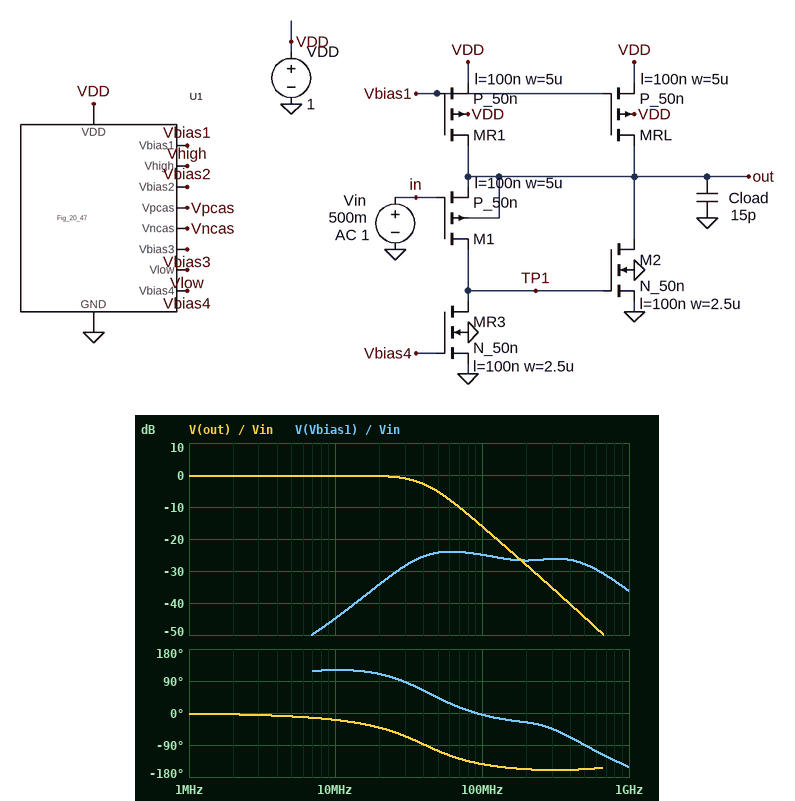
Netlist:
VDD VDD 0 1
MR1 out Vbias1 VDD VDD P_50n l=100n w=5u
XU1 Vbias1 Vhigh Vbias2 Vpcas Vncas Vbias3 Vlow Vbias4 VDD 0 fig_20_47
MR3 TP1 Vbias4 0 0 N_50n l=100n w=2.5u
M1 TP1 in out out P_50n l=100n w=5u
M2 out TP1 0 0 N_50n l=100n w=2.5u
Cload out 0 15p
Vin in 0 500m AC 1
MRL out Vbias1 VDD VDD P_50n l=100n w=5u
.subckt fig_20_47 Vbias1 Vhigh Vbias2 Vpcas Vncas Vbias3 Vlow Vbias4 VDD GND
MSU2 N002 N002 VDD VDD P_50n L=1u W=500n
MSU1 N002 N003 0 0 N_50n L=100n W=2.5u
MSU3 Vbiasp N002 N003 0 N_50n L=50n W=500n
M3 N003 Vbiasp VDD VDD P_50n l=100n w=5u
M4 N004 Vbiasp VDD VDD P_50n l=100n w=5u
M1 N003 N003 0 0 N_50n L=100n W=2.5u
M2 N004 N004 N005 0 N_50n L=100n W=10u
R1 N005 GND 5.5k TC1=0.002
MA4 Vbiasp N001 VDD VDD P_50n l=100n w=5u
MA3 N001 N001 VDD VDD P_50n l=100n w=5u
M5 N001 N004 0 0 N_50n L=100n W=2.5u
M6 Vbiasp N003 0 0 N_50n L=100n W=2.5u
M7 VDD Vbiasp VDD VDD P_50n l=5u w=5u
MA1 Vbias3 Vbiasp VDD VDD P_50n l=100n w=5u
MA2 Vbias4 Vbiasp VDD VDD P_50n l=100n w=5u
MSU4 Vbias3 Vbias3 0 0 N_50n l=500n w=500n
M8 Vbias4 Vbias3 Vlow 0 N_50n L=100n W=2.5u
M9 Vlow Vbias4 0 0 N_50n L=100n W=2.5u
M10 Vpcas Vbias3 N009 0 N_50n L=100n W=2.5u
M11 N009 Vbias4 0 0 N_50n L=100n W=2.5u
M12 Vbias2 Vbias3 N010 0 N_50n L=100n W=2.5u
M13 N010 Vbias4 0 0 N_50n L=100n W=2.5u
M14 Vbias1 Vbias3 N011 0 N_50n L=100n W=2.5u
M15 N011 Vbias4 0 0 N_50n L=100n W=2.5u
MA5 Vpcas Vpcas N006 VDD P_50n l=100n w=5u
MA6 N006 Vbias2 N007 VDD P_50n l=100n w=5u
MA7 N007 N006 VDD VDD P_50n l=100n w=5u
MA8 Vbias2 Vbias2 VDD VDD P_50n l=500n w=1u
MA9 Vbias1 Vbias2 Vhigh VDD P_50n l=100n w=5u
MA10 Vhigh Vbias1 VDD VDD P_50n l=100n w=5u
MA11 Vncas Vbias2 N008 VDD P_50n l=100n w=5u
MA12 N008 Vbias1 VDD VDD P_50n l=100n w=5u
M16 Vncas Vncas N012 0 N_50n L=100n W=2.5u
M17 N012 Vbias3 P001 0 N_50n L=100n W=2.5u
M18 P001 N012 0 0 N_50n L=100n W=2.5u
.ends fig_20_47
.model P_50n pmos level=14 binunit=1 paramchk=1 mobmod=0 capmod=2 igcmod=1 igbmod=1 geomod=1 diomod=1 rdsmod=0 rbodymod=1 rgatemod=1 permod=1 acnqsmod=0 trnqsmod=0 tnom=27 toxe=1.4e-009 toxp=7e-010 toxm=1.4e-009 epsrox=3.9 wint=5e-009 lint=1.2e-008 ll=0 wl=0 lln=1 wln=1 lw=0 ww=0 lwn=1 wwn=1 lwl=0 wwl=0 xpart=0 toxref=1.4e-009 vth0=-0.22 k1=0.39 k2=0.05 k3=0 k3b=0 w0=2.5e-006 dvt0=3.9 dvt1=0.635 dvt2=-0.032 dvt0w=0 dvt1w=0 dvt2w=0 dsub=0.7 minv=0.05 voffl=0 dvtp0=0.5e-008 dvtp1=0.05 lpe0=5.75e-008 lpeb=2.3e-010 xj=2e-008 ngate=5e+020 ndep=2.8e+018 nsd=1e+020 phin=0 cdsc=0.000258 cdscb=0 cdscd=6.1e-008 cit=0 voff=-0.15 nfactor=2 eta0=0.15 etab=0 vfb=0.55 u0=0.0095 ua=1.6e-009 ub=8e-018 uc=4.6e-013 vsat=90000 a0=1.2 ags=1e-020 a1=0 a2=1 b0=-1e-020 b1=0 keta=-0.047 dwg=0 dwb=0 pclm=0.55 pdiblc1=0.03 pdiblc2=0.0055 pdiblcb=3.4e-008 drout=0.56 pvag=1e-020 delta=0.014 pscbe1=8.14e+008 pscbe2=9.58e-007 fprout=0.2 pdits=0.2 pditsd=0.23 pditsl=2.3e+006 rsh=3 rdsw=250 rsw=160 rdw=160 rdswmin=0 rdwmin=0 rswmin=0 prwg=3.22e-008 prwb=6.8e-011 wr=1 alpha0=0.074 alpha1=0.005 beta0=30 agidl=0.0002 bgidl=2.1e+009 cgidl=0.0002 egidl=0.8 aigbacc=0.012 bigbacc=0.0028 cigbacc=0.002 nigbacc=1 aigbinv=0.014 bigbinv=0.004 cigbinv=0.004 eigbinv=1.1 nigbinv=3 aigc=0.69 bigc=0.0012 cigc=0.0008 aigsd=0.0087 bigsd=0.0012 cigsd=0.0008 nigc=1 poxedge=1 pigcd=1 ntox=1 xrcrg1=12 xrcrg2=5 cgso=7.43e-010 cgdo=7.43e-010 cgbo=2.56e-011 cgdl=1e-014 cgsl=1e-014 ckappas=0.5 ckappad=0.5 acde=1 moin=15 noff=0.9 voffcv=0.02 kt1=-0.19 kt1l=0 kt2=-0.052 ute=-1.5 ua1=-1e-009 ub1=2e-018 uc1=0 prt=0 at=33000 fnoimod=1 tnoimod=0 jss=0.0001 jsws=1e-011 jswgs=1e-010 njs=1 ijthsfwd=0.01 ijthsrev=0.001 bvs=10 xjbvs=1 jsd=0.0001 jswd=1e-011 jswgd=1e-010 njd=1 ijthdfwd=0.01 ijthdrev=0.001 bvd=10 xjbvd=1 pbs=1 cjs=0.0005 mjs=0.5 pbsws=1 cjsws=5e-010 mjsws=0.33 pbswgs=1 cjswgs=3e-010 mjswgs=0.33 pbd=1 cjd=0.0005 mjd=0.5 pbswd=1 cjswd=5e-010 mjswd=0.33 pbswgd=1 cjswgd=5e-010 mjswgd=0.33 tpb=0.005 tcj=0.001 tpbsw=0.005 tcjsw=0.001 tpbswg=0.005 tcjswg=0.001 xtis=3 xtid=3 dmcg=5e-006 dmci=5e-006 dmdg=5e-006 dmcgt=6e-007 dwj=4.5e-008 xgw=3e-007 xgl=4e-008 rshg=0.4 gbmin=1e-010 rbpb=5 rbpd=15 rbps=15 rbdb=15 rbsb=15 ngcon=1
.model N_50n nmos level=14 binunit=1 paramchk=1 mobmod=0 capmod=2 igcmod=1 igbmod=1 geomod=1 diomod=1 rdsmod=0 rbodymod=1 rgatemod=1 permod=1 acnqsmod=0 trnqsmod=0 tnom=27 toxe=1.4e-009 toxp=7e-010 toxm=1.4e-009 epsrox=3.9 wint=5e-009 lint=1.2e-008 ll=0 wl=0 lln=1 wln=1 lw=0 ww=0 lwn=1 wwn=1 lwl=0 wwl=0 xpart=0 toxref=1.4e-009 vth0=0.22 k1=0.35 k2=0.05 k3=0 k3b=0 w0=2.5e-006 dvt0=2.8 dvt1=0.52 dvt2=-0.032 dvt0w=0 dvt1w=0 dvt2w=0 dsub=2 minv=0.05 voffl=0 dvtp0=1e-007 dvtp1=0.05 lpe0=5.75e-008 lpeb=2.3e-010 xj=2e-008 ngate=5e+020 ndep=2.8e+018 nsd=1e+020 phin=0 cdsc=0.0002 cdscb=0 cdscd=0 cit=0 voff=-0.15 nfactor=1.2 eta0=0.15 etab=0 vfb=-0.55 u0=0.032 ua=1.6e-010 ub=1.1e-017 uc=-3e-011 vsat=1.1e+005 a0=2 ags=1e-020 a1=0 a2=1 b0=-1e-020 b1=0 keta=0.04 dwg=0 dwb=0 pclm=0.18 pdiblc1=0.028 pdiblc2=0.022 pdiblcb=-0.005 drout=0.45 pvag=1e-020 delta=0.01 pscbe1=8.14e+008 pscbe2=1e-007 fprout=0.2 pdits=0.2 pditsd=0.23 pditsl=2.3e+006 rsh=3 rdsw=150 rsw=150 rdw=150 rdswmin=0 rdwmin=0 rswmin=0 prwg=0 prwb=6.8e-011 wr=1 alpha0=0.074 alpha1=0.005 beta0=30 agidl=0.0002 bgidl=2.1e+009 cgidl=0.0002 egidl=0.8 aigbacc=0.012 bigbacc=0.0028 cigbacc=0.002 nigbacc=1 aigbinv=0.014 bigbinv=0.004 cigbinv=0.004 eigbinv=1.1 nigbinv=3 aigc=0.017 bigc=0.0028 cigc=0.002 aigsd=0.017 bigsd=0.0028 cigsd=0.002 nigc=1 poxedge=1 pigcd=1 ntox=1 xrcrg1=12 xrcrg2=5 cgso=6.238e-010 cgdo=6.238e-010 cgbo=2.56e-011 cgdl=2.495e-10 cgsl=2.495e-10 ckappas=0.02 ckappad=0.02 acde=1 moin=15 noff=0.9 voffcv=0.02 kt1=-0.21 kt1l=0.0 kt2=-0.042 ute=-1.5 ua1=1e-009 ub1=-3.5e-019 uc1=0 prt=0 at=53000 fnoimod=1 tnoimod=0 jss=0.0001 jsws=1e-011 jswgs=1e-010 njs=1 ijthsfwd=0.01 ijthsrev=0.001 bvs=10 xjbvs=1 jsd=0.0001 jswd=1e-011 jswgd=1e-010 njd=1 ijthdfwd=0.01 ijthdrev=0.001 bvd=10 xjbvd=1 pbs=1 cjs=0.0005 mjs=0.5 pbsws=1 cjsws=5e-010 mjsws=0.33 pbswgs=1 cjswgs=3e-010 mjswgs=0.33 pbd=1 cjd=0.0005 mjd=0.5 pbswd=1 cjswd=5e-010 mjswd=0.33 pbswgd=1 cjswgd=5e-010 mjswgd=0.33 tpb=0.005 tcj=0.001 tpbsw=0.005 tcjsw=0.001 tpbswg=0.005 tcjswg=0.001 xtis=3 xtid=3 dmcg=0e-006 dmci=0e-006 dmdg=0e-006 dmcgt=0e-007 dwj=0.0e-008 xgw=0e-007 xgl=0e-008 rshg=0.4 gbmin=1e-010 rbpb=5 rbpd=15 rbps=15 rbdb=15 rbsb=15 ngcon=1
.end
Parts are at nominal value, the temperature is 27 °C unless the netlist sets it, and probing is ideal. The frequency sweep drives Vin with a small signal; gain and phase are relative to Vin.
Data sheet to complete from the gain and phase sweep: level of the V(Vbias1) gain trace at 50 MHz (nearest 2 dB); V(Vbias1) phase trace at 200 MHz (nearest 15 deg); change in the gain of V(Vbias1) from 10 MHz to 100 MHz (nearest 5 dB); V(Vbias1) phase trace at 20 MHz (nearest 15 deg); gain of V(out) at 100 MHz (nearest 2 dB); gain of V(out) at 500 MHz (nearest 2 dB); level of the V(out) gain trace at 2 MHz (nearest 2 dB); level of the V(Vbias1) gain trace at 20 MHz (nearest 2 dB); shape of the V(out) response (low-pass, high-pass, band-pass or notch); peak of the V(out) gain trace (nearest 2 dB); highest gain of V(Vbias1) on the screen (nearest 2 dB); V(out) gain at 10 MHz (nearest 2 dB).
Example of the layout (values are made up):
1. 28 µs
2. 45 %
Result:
1. -24 dB
2. -30 deg
3. 20 dB
4. 105 deg
5. -16 dB
6. -44 dB
7. 0 dB
8. -34 dB
9. low-pass
10. 0 dB
11. -24 dB
12. 0 dB
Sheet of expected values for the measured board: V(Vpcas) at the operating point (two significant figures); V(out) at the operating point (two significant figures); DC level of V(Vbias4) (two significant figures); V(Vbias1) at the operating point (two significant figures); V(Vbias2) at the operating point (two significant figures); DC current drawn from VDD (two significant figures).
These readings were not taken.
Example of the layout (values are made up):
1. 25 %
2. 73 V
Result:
1. 200 mV
2. 860 mV
3. 360 mV
4. 640 mV
5. 370 mV
6. 130 µA
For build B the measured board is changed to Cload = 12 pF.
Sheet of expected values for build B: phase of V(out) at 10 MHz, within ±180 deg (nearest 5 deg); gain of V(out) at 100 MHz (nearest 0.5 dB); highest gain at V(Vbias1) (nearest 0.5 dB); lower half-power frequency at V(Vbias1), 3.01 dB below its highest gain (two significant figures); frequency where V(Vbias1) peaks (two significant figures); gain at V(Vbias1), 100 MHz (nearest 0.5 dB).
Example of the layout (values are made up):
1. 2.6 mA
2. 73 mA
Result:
1. -15 deg
2. -14.0 dB
3. -23.5 dB
4. 36 MHz
5. 62 MHz
6. -24.5 dB
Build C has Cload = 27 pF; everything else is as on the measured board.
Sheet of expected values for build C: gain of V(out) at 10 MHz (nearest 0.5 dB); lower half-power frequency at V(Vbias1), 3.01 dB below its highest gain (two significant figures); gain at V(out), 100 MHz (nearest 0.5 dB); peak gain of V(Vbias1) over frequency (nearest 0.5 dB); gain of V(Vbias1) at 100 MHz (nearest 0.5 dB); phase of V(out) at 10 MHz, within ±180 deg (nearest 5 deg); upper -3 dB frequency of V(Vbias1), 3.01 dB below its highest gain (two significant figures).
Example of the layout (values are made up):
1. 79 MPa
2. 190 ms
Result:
1. -1.0 dB
2. 29 MHz
3. -21.5 dB
4. -25.0 dB
5. -25.5 dB
6. -35 deg
7. 500 MHz
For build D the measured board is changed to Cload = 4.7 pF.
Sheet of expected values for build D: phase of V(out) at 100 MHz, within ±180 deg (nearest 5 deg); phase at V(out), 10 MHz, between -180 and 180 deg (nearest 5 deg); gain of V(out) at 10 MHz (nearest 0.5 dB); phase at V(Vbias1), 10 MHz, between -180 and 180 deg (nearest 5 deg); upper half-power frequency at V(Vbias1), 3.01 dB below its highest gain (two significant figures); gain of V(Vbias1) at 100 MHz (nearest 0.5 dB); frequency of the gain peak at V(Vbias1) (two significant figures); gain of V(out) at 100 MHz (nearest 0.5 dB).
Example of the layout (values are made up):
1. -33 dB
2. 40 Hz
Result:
1. -125 deg
2. -5 deg
3. 0 dB
4. 105 deg
5. 140 MHz
6. -21.5 dB
7. 79 MHz
8. -4.0 dB
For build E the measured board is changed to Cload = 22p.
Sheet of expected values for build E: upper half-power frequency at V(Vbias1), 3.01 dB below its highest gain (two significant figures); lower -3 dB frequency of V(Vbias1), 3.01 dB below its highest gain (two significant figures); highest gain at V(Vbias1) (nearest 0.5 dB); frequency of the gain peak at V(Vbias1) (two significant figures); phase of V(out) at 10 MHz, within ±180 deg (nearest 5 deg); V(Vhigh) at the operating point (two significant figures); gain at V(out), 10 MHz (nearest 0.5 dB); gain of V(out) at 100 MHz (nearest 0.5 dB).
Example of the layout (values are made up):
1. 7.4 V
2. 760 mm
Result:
1. 480 MHz
2. 30 MHz
3. -24.5 dB
4. 63 MHz
5. -30 deg
6. 790 mV
7. -0.5 dB
8. -20.0 dB
